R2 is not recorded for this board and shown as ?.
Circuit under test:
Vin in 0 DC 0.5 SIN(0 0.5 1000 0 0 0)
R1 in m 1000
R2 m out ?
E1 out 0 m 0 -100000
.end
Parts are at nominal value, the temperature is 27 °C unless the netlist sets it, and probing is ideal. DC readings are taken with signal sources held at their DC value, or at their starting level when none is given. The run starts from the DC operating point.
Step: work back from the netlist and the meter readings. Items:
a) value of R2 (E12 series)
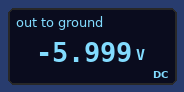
12 kΩ
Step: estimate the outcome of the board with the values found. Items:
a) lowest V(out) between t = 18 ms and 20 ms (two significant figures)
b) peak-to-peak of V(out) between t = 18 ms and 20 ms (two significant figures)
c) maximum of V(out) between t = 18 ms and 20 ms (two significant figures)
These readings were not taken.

-6.0 V
12 V
6.0 V
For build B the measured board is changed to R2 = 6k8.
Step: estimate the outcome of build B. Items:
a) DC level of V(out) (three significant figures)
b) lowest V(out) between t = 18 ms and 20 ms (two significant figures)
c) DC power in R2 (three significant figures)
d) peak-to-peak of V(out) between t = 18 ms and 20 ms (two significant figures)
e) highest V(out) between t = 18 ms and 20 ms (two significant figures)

-3.40 V
-3.4 V
1.70 mW
6.8 V
3.4 V
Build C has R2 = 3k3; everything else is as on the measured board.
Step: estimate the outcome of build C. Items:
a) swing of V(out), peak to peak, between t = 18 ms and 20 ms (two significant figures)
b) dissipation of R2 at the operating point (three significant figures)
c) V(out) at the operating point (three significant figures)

3.3 V
825 µW
-1.65 V
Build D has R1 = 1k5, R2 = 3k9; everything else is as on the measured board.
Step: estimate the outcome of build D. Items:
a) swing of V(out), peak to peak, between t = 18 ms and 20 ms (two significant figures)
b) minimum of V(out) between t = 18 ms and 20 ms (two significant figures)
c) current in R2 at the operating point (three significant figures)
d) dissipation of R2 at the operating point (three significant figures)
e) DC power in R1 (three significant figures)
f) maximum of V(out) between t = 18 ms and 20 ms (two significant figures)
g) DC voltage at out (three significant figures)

2.6 V
-1.3 V
333 µA
433 µW
167 µW
1.3 V
-1.30 V
